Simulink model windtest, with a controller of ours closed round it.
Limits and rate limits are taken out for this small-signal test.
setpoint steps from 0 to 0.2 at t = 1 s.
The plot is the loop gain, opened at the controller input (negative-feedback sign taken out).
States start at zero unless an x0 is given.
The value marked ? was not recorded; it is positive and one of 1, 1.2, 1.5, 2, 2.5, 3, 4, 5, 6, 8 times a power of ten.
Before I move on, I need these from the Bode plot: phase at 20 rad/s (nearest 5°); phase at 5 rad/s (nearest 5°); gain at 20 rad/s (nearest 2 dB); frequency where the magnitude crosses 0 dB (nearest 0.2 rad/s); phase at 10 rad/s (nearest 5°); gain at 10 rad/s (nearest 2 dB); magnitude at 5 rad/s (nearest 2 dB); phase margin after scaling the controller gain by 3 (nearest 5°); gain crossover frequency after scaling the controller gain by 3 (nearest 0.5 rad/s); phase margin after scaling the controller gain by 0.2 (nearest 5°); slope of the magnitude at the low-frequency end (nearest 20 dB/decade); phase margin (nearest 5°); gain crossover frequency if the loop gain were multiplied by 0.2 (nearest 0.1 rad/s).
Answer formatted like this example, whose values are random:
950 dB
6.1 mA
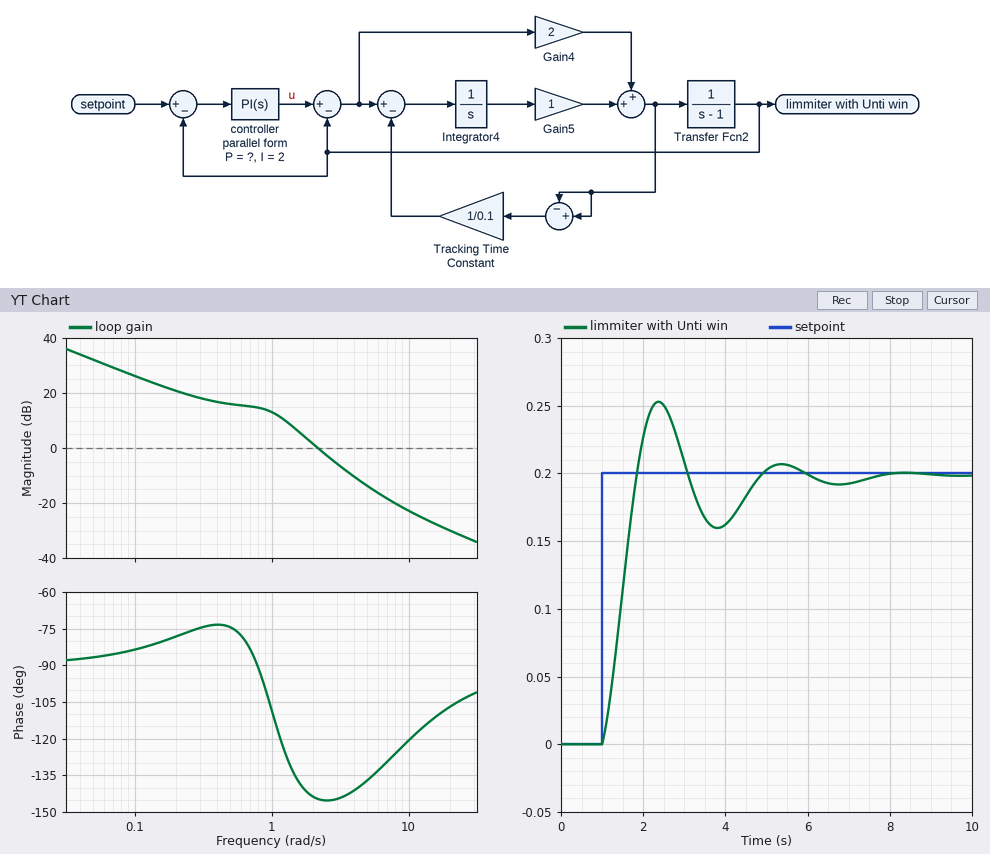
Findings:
-105°
-135°
-30 dB
2.2 rad/s
-120°
-22 dB
-14 dB
40°
4.0 rad/s
80°
-20 dB/decade
35°
0.9 rad/s
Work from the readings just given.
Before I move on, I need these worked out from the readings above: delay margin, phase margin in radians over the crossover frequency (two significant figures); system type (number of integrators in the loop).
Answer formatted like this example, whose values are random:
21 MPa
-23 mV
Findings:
0.28 s
1
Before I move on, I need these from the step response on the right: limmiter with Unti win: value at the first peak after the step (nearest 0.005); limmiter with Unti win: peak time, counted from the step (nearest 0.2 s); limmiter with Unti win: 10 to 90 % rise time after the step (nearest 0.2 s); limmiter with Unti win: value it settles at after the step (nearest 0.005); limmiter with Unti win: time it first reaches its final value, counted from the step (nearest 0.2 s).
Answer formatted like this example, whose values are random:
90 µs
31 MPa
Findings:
0.255
1.4 s
0.6 s
0.200
0.8 s
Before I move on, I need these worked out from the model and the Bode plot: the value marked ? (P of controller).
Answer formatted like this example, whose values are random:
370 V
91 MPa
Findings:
0.3
